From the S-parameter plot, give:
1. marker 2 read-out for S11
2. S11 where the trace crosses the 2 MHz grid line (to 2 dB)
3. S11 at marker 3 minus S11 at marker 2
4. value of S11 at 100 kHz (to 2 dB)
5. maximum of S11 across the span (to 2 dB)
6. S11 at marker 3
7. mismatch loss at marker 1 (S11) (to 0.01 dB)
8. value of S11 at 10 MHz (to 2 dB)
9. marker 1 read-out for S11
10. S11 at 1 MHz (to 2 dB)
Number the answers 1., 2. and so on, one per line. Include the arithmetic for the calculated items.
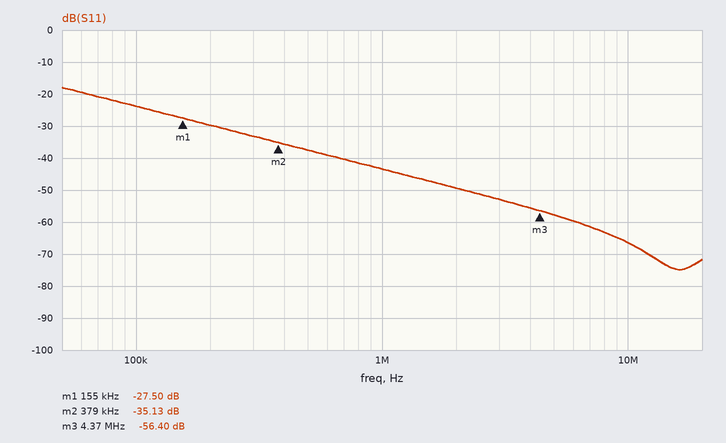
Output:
1. -35.13 dB
2. -50 dB
3. -56.4 − (-35.13) = -21.27 dB
4. -24 dB
5. -18 dB
6. -56.40 dB
7. −10 log10(1 − 10^(-27.5/10)) ≈ 0.01 dB
8. -66 dB
9. -27.50 dB
10. -44 dB
